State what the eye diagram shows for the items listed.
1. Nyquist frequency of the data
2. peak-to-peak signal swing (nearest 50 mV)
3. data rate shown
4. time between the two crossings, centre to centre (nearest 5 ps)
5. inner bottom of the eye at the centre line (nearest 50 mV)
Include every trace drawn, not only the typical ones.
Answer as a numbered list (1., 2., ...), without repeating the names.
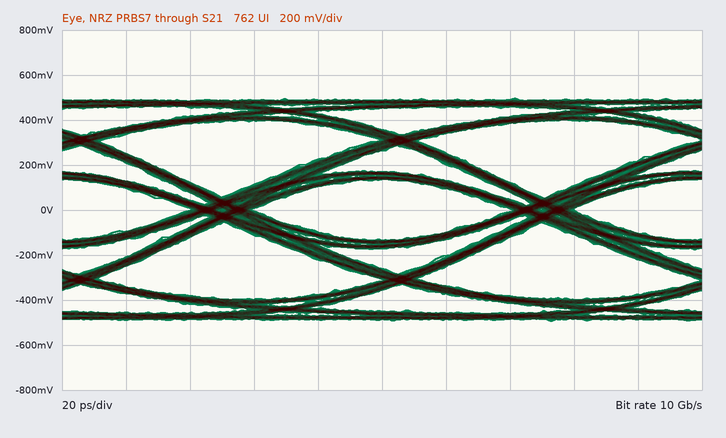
1. 5 GHz
2. 1.00 V
3. 10 Gb/s
4. 100 ps
5. -150 mV
